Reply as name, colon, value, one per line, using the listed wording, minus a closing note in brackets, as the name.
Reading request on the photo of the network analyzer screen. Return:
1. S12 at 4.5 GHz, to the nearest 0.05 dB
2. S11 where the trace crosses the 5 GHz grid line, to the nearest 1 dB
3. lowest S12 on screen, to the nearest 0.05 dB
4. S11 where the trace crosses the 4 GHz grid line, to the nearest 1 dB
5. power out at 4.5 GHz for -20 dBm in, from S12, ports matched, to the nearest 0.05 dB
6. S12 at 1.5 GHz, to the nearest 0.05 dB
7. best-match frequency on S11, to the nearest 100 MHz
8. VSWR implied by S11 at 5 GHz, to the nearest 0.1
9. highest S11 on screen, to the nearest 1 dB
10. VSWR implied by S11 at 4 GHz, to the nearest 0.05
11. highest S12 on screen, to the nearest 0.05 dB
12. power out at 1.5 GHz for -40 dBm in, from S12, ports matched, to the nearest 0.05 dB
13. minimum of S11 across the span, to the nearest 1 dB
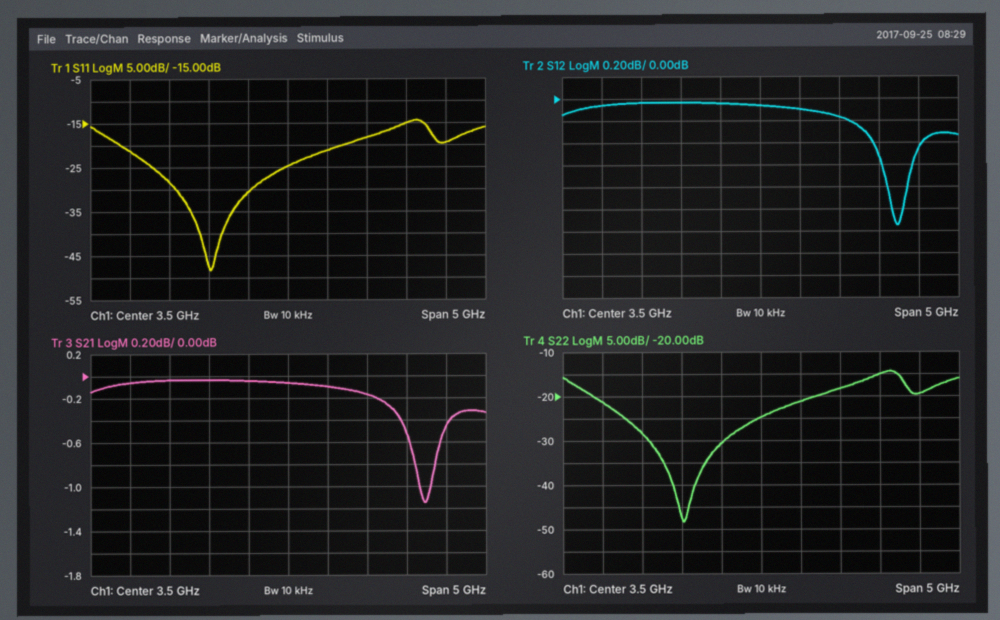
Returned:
S12 at 4.5 GHz, to the nearest 0.05 dB: -0.15 dB
S11 where the trace crosses the 5 GHz grid line, to the nearest 1 dB: -15 dB
lowest S12 on screen, to the nearest 0.05 dB: -1.15 dB
S11 where the trace crosses the 4 GHz grid line, to the nearest 1 dB: -21 dB
power out at 4.5 GHz for -20 dBm in, from S12, ports matched, to the nearest 0.05 dB: -20.15 dBm
S12 at 1.5 GHz, to the nearest 0.05 dB: -0.05 dB
best-match frequency on S11, to the nearest 100 MHz: 2.5 GHz
VSWR implied by S11 at 5 GHz, to the nearest 0.1: 1.4
highest S11 on screen, to the nearest 1 dB: -14 dB
VSWR implied by S11 at 4 GHz, to the nearest 0.05: 1.20
highest S12 on screen, to the nearest 0.05 dB: -0.05 dB
power out at 1.5 GHz for -40 dBm in, from S12, ports matched, to the nearest 0.05 dB: -40.05 dBm
minimum of S11 across the span, to the nearest 1 dB: -48 dB
